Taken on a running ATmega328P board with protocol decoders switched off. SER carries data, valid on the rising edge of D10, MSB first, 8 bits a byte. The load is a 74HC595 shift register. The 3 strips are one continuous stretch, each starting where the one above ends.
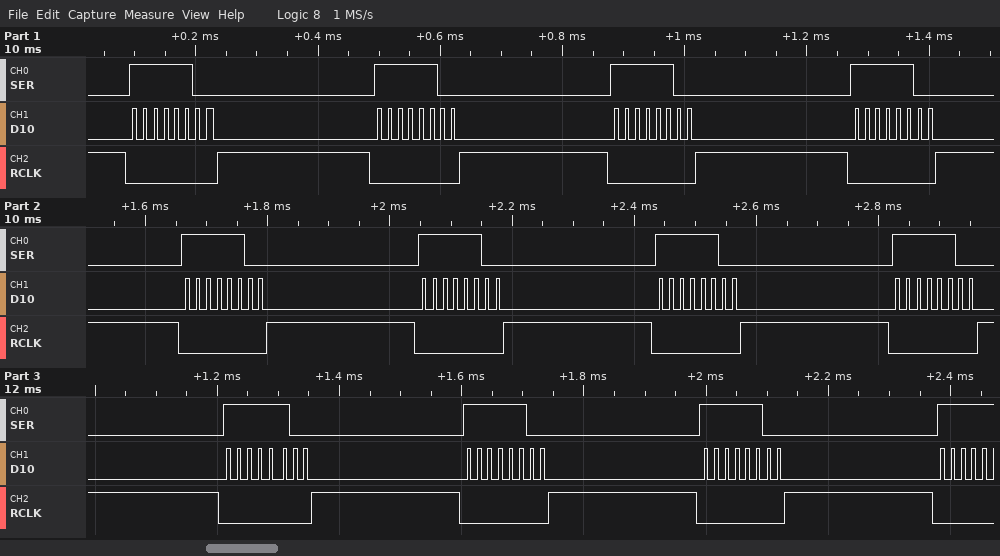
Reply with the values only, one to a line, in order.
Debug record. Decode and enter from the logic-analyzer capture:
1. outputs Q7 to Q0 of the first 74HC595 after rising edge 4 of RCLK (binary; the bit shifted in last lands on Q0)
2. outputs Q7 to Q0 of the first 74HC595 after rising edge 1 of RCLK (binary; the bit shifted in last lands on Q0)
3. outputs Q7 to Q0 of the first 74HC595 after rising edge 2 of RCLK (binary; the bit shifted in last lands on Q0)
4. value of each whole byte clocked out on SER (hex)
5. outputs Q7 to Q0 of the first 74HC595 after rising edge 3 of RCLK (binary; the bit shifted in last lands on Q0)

11111100
11111100
11111100
FC FC FC FC FC FC FC FC FC FC FC
11111100
